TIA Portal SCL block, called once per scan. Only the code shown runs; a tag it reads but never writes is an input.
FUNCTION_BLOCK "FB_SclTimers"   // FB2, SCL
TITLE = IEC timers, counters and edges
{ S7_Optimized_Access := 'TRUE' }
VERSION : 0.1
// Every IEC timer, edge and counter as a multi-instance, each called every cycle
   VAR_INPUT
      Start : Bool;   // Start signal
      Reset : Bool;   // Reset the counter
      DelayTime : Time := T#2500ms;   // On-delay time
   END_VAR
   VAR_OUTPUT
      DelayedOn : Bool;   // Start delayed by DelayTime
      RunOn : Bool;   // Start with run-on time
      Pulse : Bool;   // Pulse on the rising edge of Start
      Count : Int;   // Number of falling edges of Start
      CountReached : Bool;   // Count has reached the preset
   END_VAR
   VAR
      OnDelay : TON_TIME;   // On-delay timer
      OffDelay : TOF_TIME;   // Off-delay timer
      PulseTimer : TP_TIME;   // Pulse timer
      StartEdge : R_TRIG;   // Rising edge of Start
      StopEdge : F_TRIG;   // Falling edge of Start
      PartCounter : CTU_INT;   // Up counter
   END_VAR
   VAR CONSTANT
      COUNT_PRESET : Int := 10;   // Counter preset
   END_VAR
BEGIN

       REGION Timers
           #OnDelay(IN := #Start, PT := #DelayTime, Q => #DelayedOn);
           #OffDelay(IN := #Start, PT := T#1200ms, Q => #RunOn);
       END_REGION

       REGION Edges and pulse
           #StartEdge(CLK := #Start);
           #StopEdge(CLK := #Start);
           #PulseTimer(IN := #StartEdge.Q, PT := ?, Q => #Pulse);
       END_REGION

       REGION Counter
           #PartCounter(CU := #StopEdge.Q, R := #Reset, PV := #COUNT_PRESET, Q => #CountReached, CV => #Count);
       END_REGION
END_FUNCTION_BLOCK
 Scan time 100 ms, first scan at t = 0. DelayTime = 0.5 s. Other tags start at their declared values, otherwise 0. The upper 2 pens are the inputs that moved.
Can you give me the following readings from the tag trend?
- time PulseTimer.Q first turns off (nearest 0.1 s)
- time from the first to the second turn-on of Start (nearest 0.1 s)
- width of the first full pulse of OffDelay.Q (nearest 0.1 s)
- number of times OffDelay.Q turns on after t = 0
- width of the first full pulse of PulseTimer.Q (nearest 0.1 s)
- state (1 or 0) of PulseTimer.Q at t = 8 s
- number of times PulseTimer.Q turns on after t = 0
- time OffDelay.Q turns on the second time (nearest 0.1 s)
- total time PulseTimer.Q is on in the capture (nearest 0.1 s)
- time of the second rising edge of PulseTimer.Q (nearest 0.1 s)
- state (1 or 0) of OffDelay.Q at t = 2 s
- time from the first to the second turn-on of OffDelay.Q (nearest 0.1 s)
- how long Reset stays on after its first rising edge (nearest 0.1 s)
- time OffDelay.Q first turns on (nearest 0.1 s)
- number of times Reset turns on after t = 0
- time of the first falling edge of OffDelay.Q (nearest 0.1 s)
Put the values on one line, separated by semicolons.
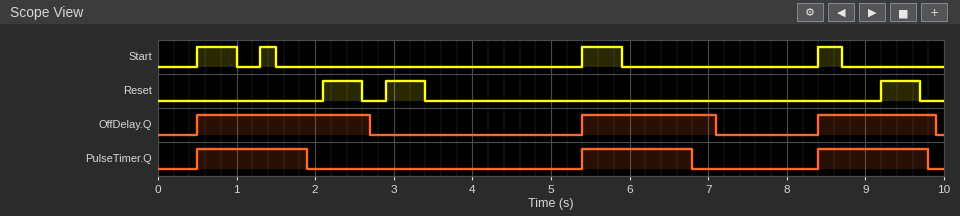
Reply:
1.9 s; 0.8 s; 2.2 s; 3; 1.4 s; 0; 3; 5.4 s; 4.2 s; 5.4 s; 1; 4.9 s; 0.5 s; 0.5 s; 3; 2.7 s
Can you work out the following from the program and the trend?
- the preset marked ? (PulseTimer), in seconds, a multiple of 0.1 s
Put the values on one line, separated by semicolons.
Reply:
1.4 s
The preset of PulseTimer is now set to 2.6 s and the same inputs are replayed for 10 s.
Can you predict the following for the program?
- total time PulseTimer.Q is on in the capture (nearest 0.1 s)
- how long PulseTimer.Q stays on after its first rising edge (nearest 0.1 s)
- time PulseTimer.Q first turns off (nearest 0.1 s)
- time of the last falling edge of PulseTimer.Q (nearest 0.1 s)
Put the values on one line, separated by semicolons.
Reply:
6.8 s; 2.6 s; 3.1 s; 8.0 s
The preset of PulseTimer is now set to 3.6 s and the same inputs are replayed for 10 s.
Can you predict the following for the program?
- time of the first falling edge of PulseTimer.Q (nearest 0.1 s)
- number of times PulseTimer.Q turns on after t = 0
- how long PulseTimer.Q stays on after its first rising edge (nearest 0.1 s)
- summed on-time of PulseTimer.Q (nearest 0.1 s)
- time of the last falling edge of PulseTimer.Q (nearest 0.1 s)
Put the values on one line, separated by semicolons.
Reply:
4.1 s; 2; 3.6 s; 7.2 s; 9.0 s
